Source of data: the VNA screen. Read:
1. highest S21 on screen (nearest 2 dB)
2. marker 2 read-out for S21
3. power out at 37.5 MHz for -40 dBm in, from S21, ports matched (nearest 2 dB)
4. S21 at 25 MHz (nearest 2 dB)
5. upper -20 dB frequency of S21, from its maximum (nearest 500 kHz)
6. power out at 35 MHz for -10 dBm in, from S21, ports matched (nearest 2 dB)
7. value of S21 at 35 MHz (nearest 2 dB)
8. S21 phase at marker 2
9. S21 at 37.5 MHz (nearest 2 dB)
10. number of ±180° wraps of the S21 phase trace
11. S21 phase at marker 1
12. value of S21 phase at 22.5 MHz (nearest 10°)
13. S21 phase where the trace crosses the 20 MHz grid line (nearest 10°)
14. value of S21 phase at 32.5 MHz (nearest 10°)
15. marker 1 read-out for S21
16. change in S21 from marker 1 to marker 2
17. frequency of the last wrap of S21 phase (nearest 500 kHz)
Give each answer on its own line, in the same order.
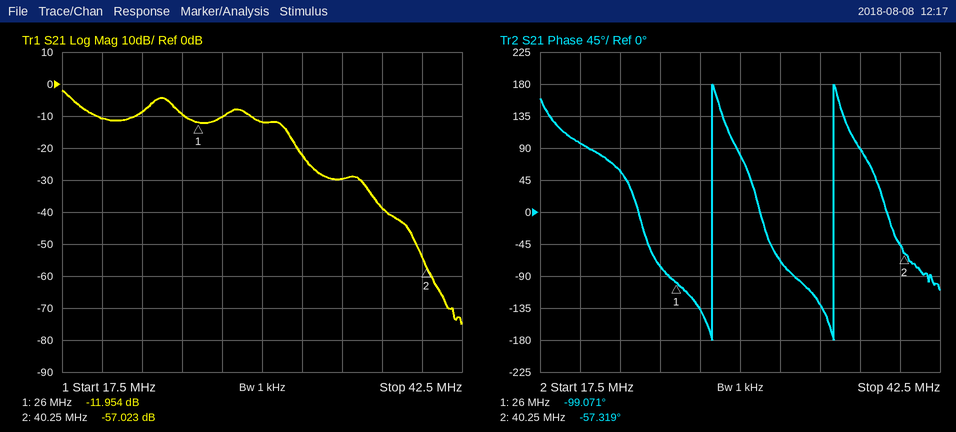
-2 dB
-57.023 dB
-78 dBm
-10 dB
32.5 MHz
-40 dBm
-30 dB
-57.319°
-38 dB
2
-99.071°
60°
100°
-70°
-11.954 dB
-45.069 dB
36.0 MHz
